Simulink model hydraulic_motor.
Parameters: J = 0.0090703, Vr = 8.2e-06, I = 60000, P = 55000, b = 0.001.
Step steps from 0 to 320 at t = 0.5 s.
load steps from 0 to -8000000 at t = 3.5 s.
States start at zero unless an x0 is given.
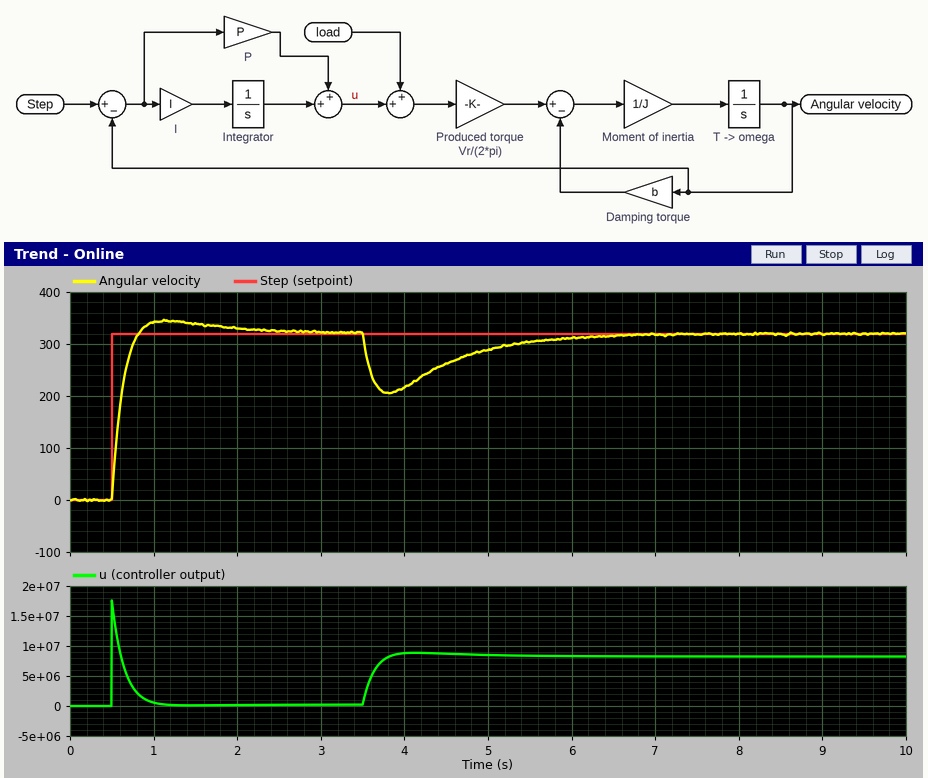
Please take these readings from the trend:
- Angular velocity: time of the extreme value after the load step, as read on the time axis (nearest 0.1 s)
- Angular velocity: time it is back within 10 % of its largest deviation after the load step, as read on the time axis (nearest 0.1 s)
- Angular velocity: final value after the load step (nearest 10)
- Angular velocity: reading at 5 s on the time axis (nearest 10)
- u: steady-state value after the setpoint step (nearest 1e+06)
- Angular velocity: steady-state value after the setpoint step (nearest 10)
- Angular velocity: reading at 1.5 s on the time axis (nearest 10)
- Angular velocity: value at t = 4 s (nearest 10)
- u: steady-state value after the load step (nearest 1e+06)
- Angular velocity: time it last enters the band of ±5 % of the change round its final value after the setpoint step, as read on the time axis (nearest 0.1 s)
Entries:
3.8 s
5.8 s
320
290
0
320
340
220
8000000
1.6 s
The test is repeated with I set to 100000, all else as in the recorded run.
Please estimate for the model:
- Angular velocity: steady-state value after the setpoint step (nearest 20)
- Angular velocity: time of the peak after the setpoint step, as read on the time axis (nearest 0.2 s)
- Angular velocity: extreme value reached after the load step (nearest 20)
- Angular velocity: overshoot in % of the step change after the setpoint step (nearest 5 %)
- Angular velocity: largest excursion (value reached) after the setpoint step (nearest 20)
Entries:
320
1.0 s
220
10 %
360
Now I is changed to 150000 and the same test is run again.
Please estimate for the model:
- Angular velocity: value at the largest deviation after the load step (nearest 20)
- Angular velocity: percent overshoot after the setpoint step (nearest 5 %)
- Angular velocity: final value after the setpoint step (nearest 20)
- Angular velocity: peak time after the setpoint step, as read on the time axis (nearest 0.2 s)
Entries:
220
15 %
320
1.0 s
